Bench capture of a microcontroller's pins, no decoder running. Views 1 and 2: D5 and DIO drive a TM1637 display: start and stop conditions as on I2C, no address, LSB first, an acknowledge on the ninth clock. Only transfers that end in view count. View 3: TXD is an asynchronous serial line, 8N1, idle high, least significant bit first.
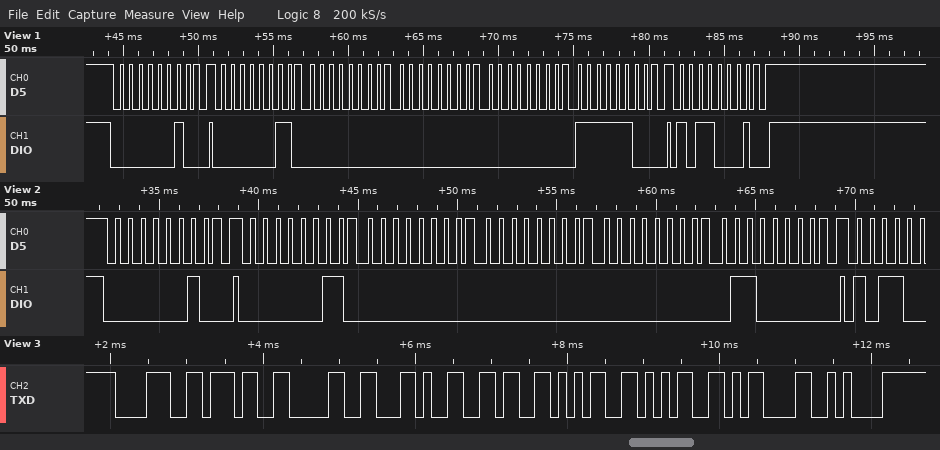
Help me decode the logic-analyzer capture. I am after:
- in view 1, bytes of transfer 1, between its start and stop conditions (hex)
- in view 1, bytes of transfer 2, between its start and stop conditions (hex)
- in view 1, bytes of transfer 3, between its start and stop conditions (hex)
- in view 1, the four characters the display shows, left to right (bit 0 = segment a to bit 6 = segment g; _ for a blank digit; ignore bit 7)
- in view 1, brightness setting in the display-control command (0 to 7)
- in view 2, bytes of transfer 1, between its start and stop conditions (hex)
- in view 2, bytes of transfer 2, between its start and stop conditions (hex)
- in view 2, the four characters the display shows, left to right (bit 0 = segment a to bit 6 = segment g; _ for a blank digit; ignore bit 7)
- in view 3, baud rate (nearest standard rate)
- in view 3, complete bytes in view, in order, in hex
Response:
40
C0 00 00 00 3F
8D
___0
5
40
C0 00 00 00 06
___1
9600 baud
38 37 30 2C 36 35 35 0D 0A
